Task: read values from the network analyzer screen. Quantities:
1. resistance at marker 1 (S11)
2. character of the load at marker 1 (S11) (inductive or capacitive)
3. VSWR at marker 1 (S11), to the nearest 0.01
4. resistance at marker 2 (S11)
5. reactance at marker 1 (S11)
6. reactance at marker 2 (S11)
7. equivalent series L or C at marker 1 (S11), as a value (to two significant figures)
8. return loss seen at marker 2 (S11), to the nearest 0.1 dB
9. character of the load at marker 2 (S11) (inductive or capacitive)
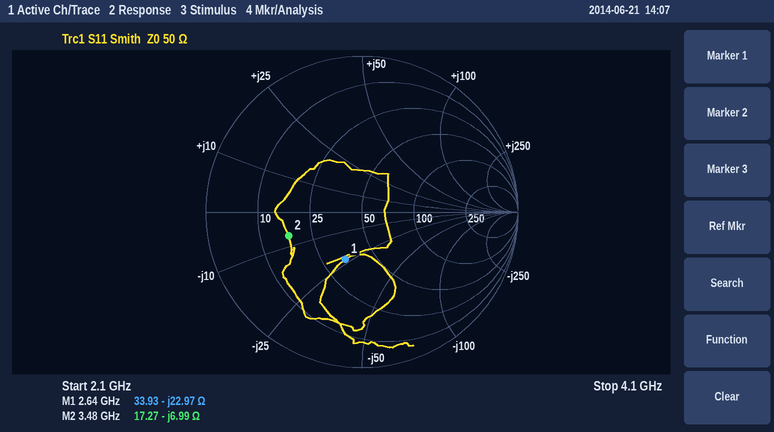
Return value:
33.93 Ω
capacitive
1.95
17.27 Ω
-22.97 Ω
-6.99 Ω
2.6 pF
6.1 dB
capacitive
